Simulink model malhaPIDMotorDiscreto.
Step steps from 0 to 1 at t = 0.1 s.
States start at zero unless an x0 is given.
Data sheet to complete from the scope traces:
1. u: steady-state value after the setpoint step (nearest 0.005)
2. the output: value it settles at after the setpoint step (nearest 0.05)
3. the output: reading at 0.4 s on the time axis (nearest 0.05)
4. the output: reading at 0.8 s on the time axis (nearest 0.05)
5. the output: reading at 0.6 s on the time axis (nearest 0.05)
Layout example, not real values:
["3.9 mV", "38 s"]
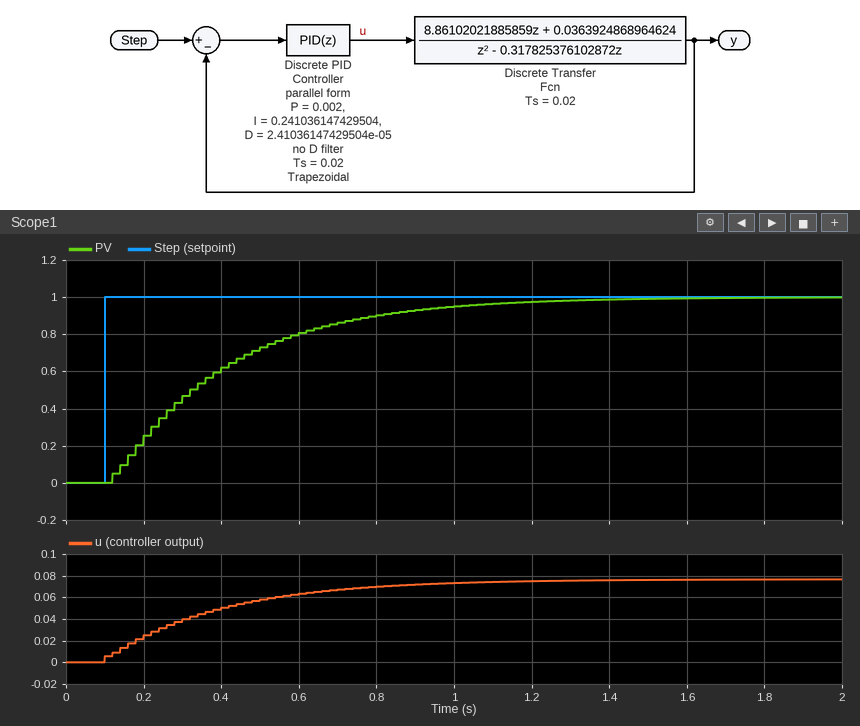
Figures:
["0.075", "1.00", "0.60", "0.90", "0.80"]
